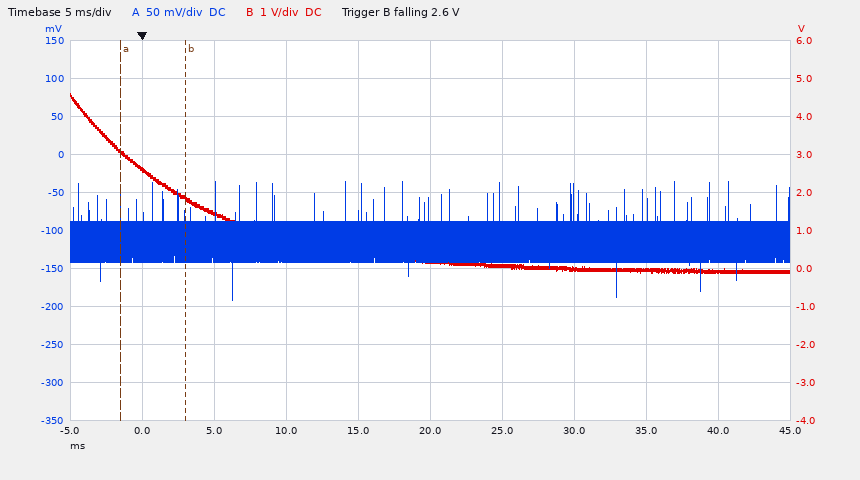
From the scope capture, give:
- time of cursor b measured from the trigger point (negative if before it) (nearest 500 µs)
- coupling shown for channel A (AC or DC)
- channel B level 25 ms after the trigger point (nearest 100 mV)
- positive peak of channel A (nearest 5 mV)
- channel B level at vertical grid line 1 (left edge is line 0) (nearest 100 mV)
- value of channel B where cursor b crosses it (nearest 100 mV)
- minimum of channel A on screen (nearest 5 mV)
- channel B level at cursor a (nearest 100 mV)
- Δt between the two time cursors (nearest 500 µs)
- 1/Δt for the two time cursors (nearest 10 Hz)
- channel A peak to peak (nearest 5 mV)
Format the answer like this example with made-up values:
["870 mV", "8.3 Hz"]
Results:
["+3.0 ms", "DC", "100 mV", "-35 mV", "2.6 V", "1.8 V", "-190 mV", "3.1 V", "4.5 ms", "220 Hz", "155 mV"]
